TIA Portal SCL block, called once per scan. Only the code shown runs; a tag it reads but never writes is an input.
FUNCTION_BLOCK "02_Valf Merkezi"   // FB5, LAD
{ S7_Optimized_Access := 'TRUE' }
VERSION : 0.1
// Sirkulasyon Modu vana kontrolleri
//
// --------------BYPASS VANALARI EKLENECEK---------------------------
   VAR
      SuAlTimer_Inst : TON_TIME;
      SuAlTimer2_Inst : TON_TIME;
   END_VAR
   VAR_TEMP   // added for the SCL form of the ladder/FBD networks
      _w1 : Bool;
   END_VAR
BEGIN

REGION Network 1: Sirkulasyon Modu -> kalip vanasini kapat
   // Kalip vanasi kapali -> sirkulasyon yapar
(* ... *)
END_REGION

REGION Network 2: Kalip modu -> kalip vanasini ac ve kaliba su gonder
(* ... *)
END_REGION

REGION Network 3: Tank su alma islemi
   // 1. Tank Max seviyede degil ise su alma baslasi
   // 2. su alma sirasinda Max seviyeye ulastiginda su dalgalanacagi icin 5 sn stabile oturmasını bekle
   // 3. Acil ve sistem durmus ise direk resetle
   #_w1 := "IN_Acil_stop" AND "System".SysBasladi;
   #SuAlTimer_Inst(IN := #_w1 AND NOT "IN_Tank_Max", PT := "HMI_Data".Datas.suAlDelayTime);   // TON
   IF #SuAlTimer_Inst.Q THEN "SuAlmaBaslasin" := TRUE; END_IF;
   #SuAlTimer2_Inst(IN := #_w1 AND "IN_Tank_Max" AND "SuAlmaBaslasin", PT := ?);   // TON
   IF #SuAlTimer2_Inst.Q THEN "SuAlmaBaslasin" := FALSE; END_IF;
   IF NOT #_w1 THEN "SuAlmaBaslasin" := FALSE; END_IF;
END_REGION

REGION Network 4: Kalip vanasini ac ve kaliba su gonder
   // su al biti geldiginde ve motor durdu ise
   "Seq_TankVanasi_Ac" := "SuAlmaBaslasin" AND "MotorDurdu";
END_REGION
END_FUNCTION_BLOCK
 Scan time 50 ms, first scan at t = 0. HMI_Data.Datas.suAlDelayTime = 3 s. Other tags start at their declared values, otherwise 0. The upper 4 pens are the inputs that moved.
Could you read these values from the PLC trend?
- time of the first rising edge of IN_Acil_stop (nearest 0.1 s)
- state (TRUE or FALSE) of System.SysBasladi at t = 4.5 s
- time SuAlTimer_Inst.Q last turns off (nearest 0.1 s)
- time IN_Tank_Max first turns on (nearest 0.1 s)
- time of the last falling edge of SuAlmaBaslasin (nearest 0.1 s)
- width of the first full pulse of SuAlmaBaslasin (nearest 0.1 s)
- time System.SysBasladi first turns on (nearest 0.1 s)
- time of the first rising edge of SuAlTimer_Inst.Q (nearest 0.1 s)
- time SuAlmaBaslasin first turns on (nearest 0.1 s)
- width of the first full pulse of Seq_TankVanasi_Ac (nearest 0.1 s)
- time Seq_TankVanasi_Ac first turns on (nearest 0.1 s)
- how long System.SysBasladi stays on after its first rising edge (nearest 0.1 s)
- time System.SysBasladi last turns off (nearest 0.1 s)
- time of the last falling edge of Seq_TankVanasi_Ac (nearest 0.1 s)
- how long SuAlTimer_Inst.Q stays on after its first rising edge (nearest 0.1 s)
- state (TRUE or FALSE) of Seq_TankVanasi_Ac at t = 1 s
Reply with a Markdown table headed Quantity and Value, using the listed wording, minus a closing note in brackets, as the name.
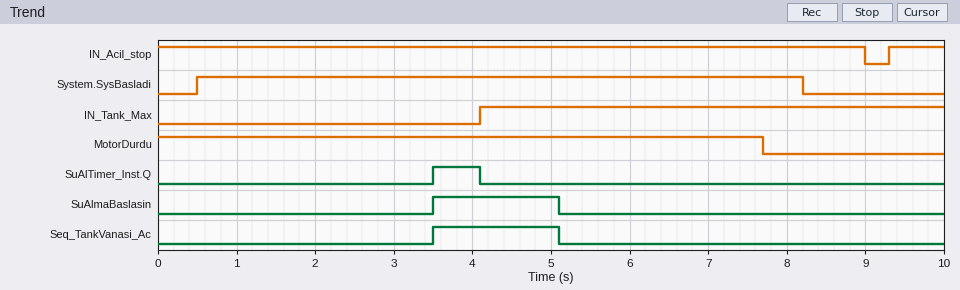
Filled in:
| Quantity | Value |
|---|---|
| time of the first rising edge of IN_Acil_stop | 9.3 s |
| state (TRUE or FALSE) of System.SysBasladi at t = 4.5 s | TRUE |
| time SuAlTimer_Inst.Q last turns off | 4.1 s |
| time IN_Tank_Max first turns on | 4.1 s |
| time of the last falling edge of SuAlmaBaslasin | 5.1 s |
| width of the first full pulse of SuAlmaBaslasin | 1.6 s |
| time System.SysBasladi first turns on | 0.5 s |
| time of the first rising edge of SuAlTimer_Inst.Q | 3.5 s |
| time SuAlmaBaslasin first turns on | 3.5 s |
| width of the first full pulse of Seq_TankVanasi_Ac | 1.6 s |
| time Seq_TankVanasi_Ac first turns on | 3.5 s |
| how long System.SysBasladi stays on after its first rising edge | 7.7 s |
| time System.SysBasladi last turns off | 8.2 s |
| time of the last falling edge of Seq_TankVanasi_Ac | 5.1 s |
| how long SuAlTimer_Inst.Q stays on after its first rising edge | 0.6 s |
| state (TRUE or FALSE) of Seq_TankVanasi_Ac at t = 1 s | FALSE |
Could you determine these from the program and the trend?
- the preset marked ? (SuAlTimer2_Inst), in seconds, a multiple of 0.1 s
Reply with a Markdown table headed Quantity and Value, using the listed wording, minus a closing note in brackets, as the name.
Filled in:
| Quantity | Value |
|---|---|
| the preset marked ? (SuAlTimer2_Inst), in seconds, a multiple of 0.1 s | 1.0 s |
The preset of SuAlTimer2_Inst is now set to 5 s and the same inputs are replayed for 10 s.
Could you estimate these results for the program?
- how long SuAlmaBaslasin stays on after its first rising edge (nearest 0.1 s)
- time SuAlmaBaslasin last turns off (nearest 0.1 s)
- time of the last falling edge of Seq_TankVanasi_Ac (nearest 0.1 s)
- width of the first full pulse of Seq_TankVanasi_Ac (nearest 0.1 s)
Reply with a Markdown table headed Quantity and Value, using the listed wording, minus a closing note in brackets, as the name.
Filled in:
| Quantity | Value |
|---|---|
| how long SuAlmaBaslasin stays on after its first rising edge | 4.7 s |
| time SuAlmaBaslasin last turns off | 8.2 s |
| time of the last falling edge of Seq_TankVanasi_Ac | 7.7 s |
| width of the first full pulse of Seq_TankVanasi_Ac | 4.2 s |
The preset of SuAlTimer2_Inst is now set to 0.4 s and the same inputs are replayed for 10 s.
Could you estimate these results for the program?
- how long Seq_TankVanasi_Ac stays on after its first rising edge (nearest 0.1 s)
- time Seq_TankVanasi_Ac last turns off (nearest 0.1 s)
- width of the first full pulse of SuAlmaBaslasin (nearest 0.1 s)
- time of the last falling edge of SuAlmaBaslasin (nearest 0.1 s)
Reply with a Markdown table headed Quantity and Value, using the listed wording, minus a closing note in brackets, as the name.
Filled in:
| Quantity | Value |
|---|---|
| how long Seq_TankVanasi_Ac stays on after its first rising edge | 1.0 s |
| time Seq_TankVanasi_Ac last turns off | 4.5 s |
| width of the first full pulse of SuAlmaBaslasin | 1.0 s |
| time of the last falling edge of SuAlmaBaslasin | 4.5 s |
